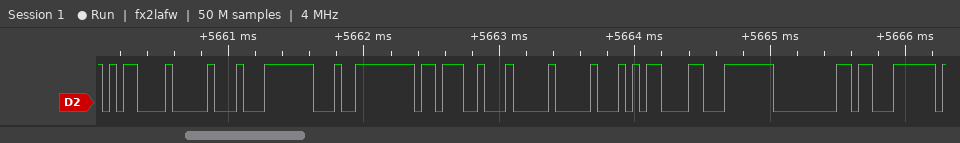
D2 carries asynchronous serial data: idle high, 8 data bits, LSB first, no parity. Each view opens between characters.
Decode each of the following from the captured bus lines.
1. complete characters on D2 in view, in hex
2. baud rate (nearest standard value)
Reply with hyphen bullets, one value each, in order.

- 0D, 10, FC, E4, 3B, 04, 10, 0D, FC, 00, E3
- 19200 baud
